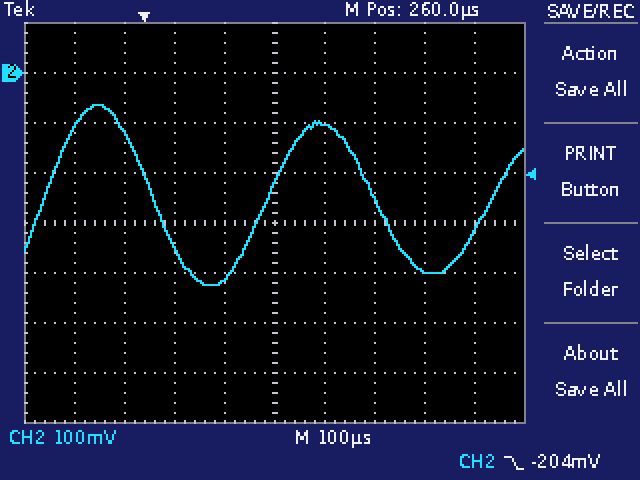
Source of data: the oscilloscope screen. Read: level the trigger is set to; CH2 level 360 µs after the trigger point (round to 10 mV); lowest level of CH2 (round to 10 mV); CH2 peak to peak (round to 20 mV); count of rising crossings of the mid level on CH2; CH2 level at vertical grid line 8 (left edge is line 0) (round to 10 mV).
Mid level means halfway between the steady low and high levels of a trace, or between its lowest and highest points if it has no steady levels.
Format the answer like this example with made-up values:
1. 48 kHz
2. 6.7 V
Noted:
1. -204 mV
2. -100 mV
3. -420 mV
4. 360 mV
5. 3
6. -400 mV
